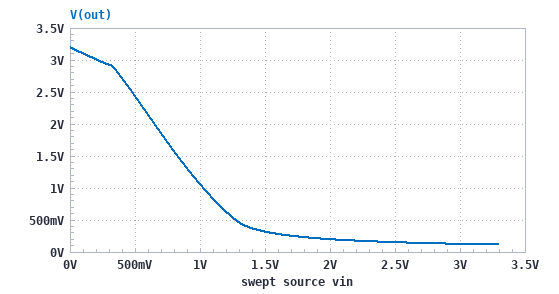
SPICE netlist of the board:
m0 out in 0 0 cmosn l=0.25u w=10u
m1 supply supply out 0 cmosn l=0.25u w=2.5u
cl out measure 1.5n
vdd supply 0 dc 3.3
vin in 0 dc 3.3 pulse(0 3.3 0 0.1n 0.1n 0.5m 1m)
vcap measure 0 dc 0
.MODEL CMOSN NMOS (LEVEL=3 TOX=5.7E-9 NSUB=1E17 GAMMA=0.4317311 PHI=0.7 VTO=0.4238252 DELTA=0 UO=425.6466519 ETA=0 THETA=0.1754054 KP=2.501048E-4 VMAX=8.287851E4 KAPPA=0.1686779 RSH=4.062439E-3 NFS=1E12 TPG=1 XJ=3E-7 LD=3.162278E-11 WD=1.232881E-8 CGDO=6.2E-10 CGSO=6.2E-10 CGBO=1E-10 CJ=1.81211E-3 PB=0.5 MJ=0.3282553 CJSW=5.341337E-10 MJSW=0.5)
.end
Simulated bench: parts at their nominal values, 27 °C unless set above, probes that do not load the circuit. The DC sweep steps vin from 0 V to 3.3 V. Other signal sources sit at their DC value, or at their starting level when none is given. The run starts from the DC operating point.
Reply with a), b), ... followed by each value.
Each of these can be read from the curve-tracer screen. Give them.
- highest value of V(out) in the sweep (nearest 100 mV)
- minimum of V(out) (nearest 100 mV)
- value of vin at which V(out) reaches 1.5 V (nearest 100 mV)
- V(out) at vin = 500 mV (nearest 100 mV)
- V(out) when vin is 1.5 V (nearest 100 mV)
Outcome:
a) 3.2 V
b) 100 mV
c) 800 mV
d) 2.4 V
e) 300 mV
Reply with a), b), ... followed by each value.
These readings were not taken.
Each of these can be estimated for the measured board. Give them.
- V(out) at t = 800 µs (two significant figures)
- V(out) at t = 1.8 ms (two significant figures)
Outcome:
a) 3.0 V
b) 3.0 V
